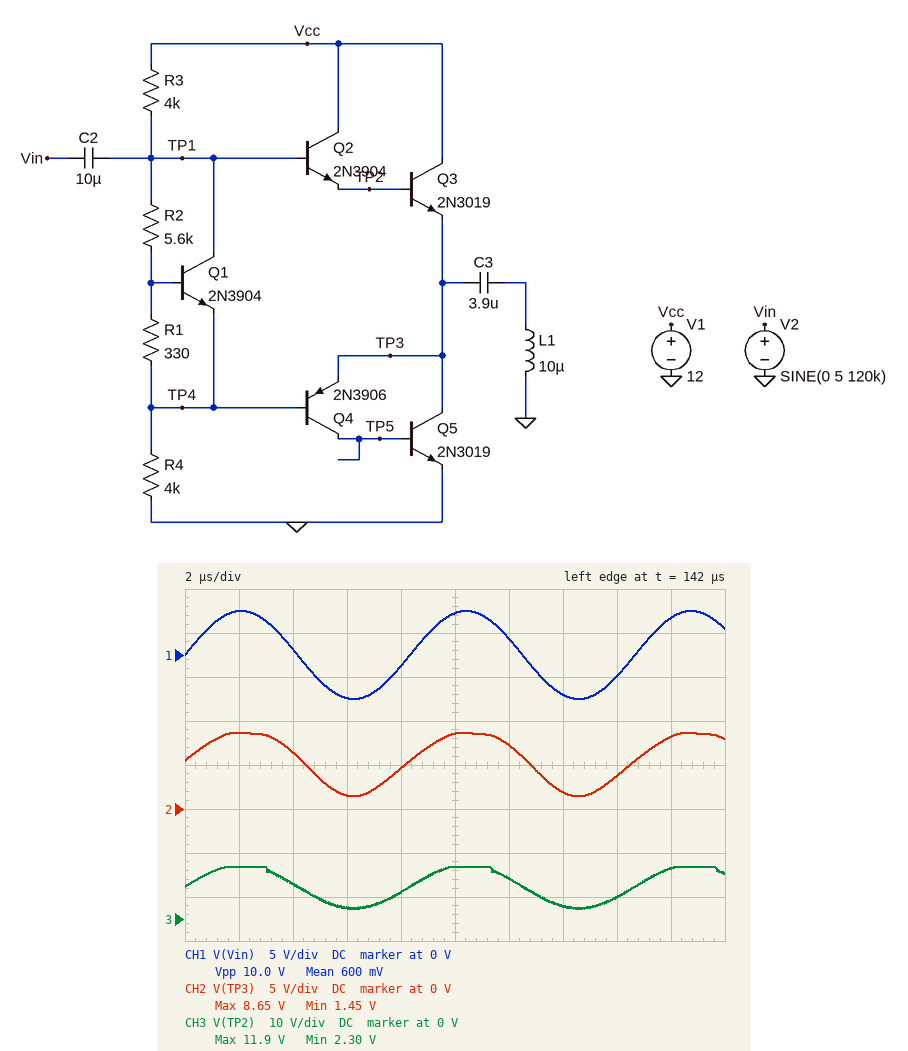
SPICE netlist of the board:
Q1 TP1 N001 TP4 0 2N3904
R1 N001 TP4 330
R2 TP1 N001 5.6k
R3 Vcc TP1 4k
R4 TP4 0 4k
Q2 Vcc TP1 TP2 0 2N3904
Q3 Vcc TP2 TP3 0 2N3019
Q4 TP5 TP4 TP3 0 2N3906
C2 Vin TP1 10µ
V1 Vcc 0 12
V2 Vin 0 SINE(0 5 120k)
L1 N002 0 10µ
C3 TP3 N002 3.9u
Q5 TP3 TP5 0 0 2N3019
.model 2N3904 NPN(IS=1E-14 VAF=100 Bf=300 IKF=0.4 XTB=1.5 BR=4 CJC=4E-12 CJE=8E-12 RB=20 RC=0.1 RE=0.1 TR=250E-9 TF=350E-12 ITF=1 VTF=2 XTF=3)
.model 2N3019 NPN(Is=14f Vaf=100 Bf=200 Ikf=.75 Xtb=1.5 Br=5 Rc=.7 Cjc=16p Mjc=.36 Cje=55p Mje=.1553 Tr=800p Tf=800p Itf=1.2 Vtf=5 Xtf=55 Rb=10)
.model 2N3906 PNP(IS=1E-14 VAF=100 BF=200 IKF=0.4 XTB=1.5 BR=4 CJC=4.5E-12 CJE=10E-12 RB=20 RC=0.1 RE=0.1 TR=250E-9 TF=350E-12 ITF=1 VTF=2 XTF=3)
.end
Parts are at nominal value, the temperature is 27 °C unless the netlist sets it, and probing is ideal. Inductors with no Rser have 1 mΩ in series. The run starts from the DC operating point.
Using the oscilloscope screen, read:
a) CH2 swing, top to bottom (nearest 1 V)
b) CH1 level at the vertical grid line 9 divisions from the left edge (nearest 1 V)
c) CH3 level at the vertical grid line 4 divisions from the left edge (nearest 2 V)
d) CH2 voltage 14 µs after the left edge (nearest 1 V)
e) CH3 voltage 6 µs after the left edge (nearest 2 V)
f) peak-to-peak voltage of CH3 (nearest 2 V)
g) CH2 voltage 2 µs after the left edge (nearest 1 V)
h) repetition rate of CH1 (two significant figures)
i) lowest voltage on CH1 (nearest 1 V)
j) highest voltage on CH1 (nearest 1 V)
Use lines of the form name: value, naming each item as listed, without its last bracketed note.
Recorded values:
CH2 swing, top to bottom: 7 V
CH1 level at the vertical grid line 9 divisions from the left edge: 4 V
CH3 level at the vertical grid line 4 divisions from the left edge: 6 V
CH2 voltage 14 µs after the left edge: 2 V
CH3 voltage 6 µs after the left edge: 2 V
peak-to-peak voltage of CH3: 10 V
CH2 voltage 2 µs after the left edge: 9 V
repetition rate of CH1: 120 kHz
lowest voltage on CH1: -5 V
highest voltage on CH1: 5 V
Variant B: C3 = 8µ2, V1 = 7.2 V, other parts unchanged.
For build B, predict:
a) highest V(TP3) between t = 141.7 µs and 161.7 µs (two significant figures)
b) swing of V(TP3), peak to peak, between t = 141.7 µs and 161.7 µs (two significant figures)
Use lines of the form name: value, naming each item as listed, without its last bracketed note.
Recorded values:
highest V(TP3) between t = 141.7 µs and 161.7 µs: 5.4 V
swing of V(TP3), peak to peak, between t = 141.7 µs and 161.7 µs: 4.5 V
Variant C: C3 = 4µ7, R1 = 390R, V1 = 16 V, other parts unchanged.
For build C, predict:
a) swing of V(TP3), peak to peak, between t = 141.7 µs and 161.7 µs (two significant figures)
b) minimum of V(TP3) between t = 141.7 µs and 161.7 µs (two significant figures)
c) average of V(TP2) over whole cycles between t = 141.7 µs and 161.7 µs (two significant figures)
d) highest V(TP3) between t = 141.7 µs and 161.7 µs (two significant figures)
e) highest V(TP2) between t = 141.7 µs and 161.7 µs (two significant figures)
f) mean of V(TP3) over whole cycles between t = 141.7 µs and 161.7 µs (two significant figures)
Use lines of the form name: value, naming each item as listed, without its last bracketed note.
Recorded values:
swing of V(TP3), peak to peak, between t = 141.7 µs and 161.7 µs: 7.4 V
minimum of V(TP3) between t = 141.7 µs and 161.7 µs: 3.6 V
average of V(TP2) over whole cycles between t = 141.7 µs and 161.7 µs: 9.9 V
highest V(TP3) between t = 141.7 µs and 161.7 µs: 11 V
highest V(TP2) between t = 141.7 µs and 161.7 µs: 15 V
mean of V(TP3) over whole cycles between t = 141.7 µs and 161.7 µs: 7.5 V
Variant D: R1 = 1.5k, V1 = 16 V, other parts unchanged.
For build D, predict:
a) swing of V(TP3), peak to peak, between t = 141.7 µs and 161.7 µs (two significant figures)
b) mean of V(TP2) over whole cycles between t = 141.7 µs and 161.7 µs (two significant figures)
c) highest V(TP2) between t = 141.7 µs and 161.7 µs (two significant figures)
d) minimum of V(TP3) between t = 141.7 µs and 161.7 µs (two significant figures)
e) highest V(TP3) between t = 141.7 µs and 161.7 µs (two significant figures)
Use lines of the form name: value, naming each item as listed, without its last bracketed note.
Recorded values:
swing of V(TP3), peak to peak, between t = 141.7 µs and 161.7 µs: 9.5 V
mean of V(TP2) over whole cycles between t = 141.7 µs and 161.7 µs: 9.0 V
highest V(TP2) between t = 141.7 µs and 161.7 µs: 14 V
minimum of V(TP3) between t = 141.7 µs and 161.7 µs: 2.9 V
highest V(TP3) between t = 141.7 µs and 161.7 µs: 12 V
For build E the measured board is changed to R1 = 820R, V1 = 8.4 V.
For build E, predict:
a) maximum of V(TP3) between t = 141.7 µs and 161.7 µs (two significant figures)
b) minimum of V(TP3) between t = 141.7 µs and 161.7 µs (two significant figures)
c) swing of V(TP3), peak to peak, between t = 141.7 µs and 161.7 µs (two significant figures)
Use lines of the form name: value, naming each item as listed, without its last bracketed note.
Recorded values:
maximum of V(TP3) between t = 141.7 µs and 161.7 µs: 6.5 V
minimum of V(TP3) between t = 141.7 µs and 161.7 µs: 950 mV
swing of V(TP3), peak to peak, between t = 141.7 µs and 161.7 µs: 5.5 V
